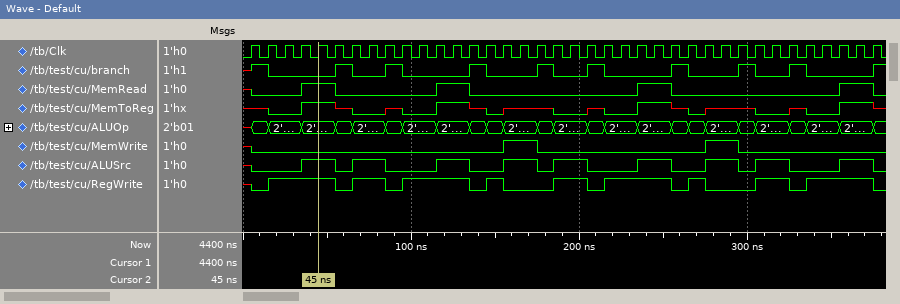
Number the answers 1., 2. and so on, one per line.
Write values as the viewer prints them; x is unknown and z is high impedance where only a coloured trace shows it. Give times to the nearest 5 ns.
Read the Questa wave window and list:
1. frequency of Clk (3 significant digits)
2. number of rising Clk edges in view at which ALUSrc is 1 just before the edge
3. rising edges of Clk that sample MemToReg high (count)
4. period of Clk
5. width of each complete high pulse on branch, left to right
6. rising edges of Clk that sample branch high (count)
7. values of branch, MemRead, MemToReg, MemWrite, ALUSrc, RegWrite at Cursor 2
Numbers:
1. 100 MHz
2. 18
3. 8
4. 10 ns
5. 10 ns, 10 ns, 10 ns, 10 ns, 10 ns, 10 ns, 10 ns, 10 ns
6. 9
7. branch=0, MemRead=1, MemToReg=1, MemWrite=0, ALUSrc=1, RegWrite=1
